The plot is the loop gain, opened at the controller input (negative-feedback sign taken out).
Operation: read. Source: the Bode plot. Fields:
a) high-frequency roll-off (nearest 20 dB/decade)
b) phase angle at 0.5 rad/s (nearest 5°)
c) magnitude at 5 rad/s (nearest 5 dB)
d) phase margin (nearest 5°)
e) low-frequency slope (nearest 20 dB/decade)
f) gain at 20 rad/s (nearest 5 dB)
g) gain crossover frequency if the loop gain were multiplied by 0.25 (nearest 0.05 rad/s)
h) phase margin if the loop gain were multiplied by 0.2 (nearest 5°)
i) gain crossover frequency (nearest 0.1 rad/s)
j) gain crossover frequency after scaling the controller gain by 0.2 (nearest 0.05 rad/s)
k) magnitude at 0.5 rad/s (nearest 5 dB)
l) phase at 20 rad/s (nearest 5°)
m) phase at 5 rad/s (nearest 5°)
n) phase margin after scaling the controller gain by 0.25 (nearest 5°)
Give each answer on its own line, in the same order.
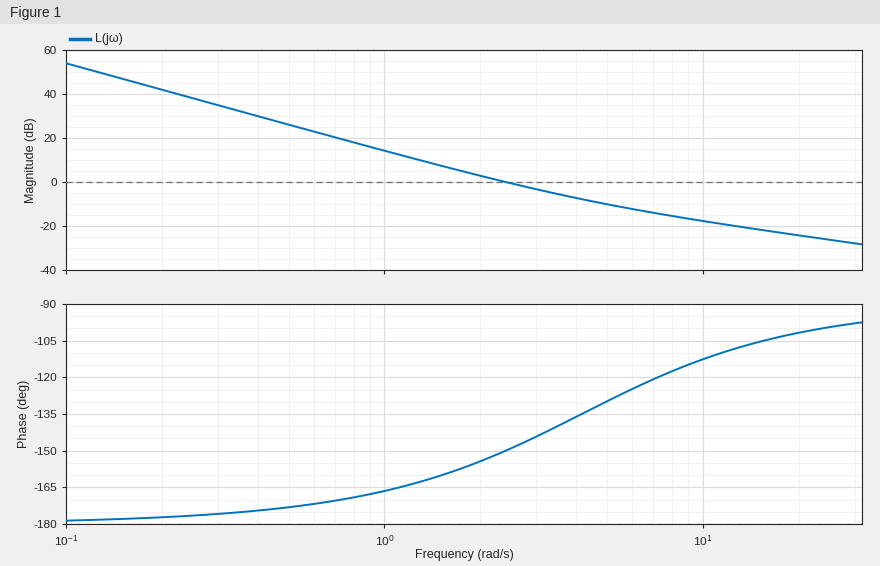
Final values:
-20 dB/decade
-175°
-10 dB
30°
-40 dB/decade
-25 dB
1.15 rad/s
15°
2.4 rad/s
1.00 rad/s
25 dB
-100°
-130°
15°
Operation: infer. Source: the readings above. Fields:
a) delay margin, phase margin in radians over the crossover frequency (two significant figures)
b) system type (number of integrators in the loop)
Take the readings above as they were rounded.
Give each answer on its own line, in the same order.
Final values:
0.22 s
2
